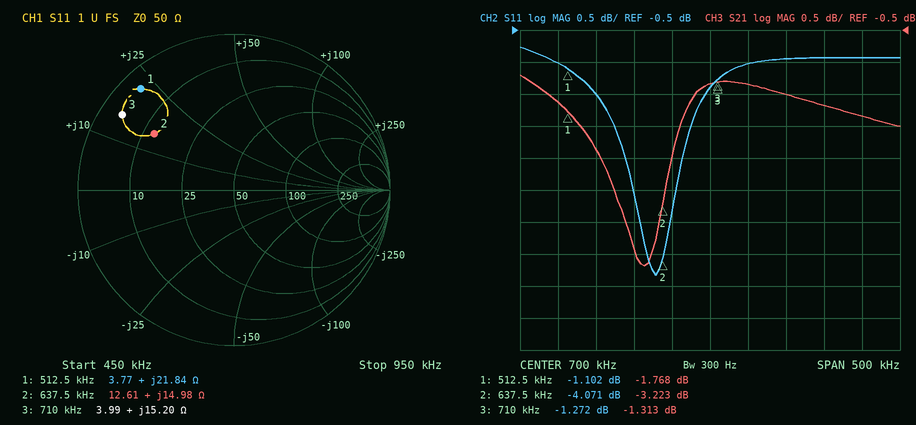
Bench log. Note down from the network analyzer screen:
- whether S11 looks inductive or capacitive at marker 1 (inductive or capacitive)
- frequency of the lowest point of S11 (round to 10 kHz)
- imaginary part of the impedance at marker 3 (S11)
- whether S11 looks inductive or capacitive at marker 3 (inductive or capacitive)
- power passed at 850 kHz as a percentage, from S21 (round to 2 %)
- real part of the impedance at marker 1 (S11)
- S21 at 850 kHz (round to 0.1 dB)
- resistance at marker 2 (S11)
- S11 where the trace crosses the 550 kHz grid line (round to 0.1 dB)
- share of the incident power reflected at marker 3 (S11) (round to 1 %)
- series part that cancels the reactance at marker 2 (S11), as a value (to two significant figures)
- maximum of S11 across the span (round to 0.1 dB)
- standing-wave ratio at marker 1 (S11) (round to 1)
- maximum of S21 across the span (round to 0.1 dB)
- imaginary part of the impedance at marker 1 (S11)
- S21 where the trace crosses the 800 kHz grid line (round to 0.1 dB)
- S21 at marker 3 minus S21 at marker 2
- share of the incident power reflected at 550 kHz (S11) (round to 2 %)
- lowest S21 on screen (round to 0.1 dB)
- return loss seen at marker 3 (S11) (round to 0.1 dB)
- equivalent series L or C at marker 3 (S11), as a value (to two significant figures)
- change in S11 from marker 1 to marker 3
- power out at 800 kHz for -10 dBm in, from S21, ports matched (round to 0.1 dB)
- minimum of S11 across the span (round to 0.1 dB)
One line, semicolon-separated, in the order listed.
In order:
inductive; 630 kHz; +15.20 Ω; inductive; 68 %; 3.77 Ω; -1.7 dB; 12.61 Ω; -1.5 dB; 75 %; 17 nF; -0.8 dB; 16; -1.2 dB; +21.84 Ω; -1.5 dB; 1.910 dB; 70 %; -4.2 dB; 1.3 dB; 3.4 µH; -0.170 dB; -11.5 dBm; -4.3 dB
